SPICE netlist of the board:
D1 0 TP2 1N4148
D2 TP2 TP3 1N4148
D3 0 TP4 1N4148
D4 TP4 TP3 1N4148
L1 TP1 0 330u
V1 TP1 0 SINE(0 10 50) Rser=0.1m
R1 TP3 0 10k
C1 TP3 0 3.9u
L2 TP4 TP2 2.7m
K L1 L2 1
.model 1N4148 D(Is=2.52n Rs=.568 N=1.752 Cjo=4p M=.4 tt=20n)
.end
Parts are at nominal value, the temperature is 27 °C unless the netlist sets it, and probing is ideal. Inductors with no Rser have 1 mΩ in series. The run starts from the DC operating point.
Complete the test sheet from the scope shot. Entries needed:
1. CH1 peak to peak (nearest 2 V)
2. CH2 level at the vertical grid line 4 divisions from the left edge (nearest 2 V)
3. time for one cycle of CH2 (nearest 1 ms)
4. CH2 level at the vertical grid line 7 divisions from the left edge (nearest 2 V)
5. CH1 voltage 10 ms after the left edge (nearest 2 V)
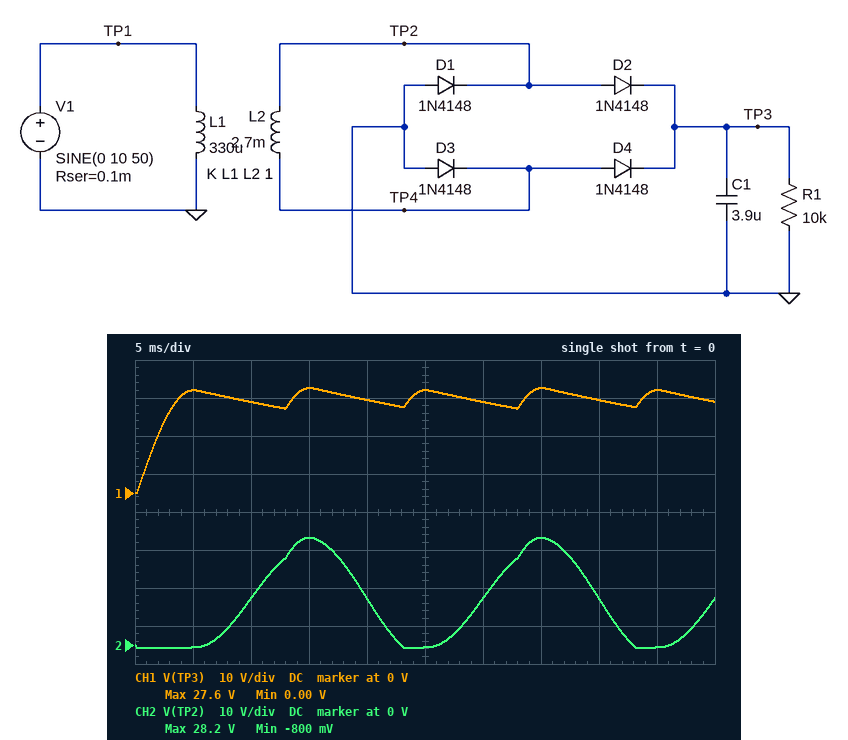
28 V
12 V
20 ms
28 V
24 V
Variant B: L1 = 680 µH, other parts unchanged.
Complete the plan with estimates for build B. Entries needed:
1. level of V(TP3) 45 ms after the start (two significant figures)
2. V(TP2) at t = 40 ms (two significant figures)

19 V
8.3 V
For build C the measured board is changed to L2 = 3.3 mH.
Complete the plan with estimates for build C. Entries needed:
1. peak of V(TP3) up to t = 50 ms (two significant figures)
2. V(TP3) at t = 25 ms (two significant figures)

31 V
30 V
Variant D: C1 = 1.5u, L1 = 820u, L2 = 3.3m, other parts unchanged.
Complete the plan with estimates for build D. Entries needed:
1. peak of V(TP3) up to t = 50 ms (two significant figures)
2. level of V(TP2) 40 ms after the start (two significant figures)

19 V
7.0 V
